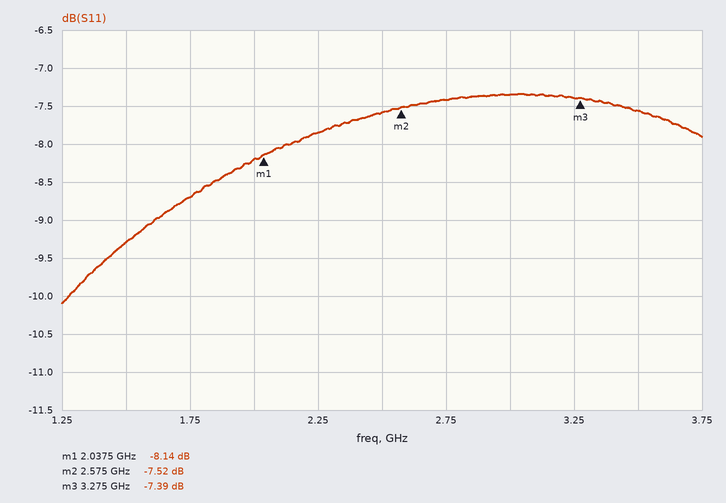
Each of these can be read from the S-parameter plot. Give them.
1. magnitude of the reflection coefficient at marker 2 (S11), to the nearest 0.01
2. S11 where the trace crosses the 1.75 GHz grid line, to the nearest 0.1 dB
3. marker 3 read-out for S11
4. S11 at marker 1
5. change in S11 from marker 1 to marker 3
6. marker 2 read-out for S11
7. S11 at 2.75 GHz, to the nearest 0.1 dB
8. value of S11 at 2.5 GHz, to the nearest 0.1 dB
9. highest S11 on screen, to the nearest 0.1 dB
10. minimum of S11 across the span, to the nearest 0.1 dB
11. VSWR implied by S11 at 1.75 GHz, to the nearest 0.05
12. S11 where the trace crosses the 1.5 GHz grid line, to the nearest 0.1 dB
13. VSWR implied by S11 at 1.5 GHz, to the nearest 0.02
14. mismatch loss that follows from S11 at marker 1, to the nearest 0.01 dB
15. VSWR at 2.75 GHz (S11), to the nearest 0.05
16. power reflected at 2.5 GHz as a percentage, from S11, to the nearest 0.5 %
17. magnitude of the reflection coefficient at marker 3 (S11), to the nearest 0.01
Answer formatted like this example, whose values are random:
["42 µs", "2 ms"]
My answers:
["0.42", "-8.7 dB", "-7.39 dB", "-8.14 dB", "0.75 dB", "-7.52 dB", "-7.4 dB", "-7.6 dB", "-7.3 dB", "-10.1 dB", "2.15", "-9.3 dB", "2.04", "0.72 dB", "2.50", "17.5 %", "0.43"]
